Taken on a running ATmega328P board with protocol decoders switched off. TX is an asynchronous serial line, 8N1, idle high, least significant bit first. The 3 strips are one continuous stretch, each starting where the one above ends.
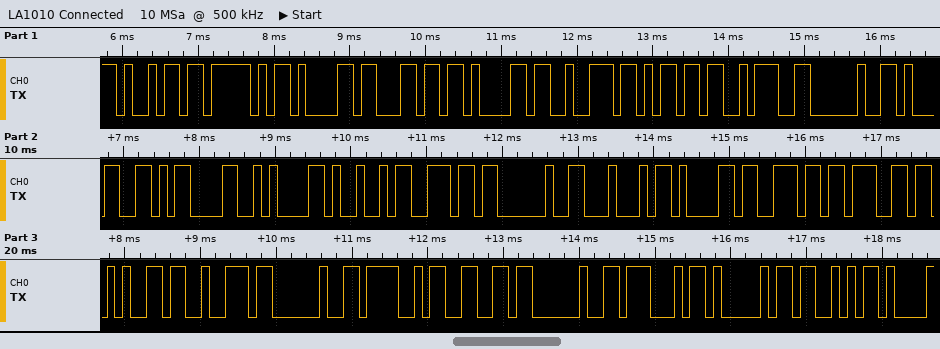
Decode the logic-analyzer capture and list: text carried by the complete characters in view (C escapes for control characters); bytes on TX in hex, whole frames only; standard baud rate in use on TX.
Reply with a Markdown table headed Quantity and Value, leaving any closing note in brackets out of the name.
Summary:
| Quantity | Value |
|---|---|
| text carried by the complete characters in view | "i_alarm: 1\r\nIn Danger Of GAS" |
| bytes on TX in hex, whole frames only | 69 5F 61 6C 61 72 6D 3A 20 31 0D 0A 49 6E 20 44 61 6E 67 65 72 20 4F 66 20 47 41 53 |
| standard baud rate in use on TX | 9600 baud |
